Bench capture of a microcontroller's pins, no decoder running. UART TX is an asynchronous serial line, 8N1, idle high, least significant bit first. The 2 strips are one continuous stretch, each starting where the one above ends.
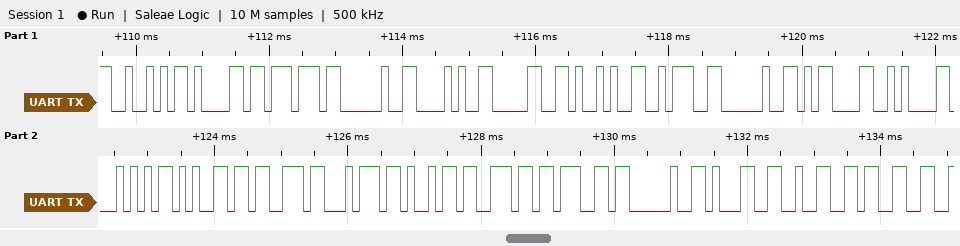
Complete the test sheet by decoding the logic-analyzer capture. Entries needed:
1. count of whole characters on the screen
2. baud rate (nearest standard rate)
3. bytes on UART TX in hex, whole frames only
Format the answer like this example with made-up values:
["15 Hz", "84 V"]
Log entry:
["22", "9600 baud", "52 61 77 20 28 30 29 3A 20 0D 0A 54 65 73 74 69 6E 67 20 31 32 33"]
